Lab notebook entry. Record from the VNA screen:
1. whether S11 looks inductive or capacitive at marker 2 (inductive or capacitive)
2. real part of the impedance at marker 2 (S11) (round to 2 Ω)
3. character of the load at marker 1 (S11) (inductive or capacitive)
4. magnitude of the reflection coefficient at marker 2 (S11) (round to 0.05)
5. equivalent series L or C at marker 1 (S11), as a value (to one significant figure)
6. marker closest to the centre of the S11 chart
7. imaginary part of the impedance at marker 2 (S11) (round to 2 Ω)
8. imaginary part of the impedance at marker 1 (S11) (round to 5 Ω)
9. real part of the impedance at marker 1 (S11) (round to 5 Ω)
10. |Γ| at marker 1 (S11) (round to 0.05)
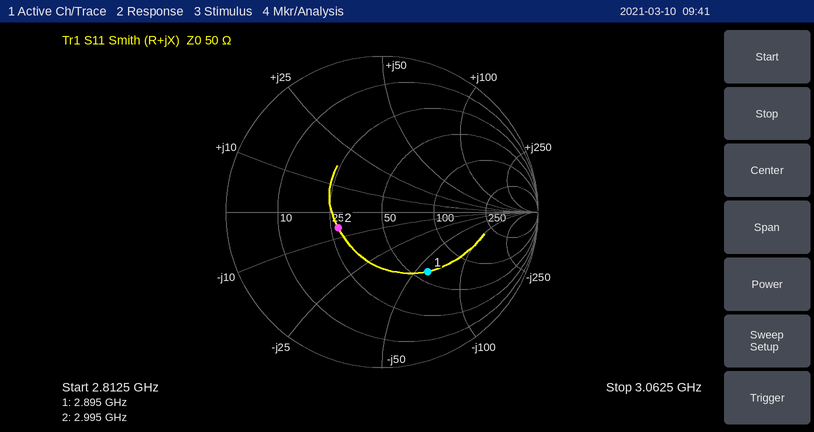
capacitive
28 Ω
capacitive
0.30
900 fF
marker 2
-6 Ω
-60 Ω
60 Ω
0.50
